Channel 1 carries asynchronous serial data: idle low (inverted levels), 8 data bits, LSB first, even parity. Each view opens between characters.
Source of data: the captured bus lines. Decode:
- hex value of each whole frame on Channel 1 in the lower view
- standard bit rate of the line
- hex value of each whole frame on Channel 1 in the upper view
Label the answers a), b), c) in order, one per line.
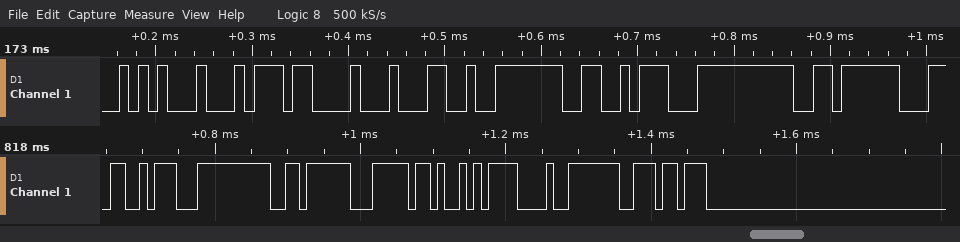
a) 16, 00, 02, 90, 85, 03, 24
b) 100000 baud
c) 75, 91, 77, 03, 16, 00, 02
